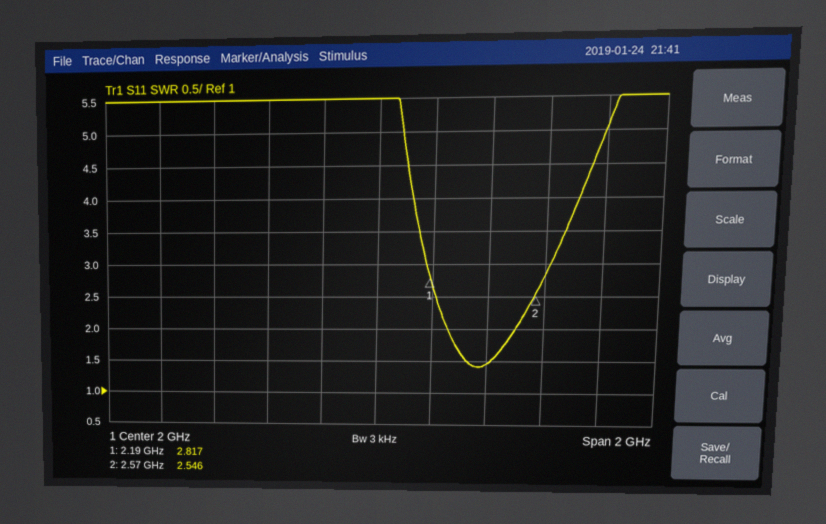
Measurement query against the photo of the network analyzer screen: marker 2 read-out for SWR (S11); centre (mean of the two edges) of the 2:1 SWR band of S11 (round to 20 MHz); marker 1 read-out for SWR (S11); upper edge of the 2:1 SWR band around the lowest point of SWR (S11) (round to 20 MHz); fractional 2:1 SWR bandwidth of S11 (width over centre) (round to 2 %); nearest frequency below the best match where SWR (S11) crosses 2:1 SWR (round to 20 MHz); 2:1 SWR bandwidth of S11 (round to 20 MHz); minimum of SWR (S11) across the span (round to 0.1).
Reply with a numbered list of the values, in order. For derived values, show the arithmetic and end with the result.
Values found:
1. 2.546
2. 2.38 GHz
3. 2.817
4. 2.50 GHz
5. 240 MHz / 2.38 GHz ≈ 10 %
6. 2.26 GHz
7. 2.50 GHz − 2.26 GHz = 240 MHz
8. 1.4
